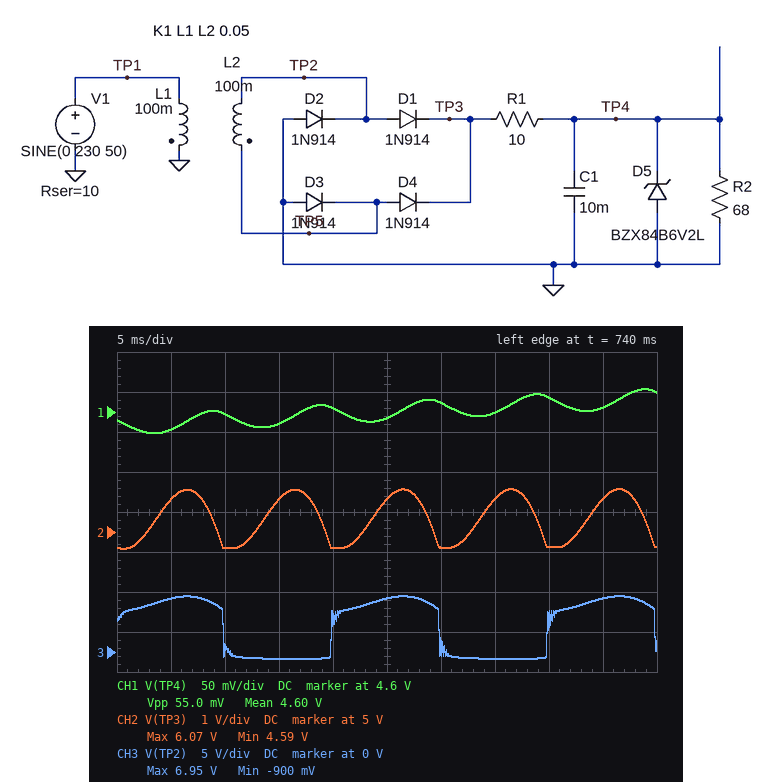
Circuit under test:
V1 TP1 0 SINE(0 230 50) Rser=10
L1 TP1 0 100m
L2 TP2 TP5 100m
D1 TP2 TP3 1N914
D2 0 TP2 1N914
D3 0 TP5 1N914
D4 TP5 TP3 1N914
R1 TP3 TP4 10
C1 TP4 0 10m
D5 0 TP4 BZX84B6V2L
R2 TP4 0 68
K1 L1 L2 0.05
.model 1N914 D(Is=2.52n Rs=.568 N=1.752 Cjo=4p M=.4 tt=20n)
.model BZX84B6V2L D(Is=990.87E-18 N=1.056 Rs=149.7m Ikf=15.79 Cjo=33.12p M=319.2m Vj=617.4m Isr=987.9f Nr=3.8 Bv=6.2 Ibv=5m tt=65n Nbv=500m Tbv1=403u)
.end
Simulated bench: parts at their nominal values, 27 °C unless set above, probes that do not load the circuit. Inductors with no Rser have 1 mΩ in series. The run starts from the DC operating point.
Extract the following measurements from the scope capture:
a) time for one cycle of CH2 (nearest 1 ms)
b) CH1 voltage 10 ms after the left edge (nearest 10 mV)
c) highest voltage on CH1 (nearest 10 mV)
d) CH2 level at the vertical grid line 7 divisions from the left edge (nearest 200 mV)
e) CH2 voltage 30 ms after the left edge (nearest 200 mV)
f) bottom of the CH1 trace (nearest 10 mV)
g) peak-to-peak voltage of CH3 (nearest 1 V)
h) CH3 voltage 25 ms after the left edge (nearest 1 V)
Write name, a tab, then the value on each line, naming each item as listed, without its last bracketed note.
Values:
time for one cycle of CH2	10 ms
CH1 voltage 10 ms after the left edge	4.60 V
highest voltage on CH1	4.63 V
CH2 level at the vertical grid line 7 divisions from the left edge	5.8 V
CH2 voltage 30 ms after the left edge	4.6 V
bottom of the CH1 trace	4.57 V
peak-to-peak voltage of CH3	8 V
CH3 voltage 25 ms after the left edge	7 V
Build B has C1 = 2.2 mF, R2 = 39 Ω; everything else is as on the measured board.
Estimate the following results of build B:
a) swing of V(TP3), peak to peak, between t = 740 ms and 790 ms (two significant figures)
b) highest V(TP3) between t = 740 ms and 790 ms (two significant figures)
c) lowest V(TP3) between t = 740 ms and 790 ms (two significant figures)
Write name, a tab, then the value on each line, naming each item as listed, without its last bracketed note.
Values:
swing of V(TP3), peak to peak, between t = 740 ms and 790 ms	1.8 V
highest V(TP3) between t = 740 ms and 790 ms	5.6 V
lowest V(TP3) between t = 740 ms and 790 ms	3.9 V
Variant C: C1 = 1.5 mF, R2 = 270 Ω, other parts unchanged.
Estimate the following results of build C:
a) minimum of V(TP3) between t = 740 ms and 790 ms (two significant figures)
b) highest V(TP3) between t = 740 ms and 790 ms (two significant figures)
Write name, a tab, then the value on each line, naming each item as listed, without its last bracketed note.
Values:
minimum of V(TP3) between t = 740 ms and 790 ms	6.2 V
highest V(TP3) between t = 740 ms and 790 ms	7.1 V
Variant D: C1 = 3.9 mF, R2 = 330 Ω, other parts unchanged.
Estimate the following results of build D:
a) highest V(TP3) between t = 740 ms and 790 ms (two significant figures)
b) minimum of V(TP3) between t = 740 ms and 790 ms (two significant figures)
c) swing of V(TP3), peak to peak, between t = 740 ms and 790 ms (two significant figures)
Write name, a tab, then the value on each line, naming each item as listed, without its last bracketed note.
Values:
highest V(TP3) between t = 740 ms and 790 ms	7.1 V
minimum of V(TP3) between t = 740 ms and 790 ms	6.2 V
swing of V(TP3), peak to peak, between t = 740 ms and 790 ms	870 mV
